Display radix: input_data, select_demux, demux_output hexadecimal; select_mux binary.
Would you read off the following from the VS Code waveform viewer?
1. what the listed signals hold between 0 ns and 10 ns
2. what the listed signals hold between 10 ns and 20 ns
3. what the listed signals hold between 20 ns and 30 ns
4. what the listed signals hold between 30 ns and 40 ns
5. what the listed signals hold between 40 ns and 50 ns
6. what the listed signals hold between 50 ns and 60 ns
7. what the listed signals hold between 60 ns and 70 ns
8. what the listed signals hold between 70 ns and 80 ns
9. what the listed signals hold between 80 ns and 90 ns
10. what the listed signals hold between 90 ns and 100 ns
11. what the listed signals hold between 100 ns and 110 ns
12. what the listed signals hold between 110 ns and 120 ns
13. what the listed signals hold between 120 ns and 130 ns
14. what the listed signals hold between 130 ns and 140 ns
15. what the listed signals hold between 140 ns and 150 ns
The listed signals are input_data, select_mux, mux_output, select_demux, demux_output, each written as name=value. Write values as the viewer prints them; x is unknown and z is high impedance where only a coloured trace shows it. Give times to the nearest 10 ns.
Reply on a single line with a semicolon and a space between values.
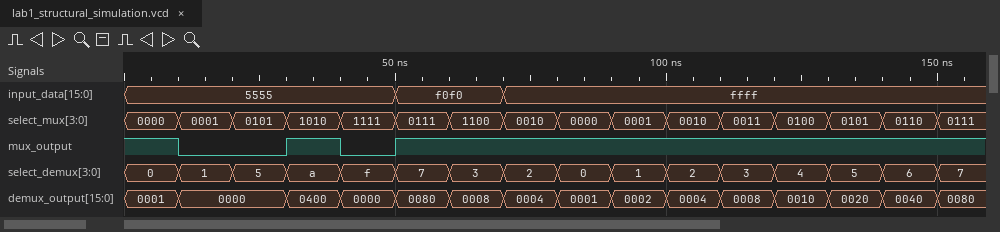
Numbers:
input_data=5555, select_mux=0000, mux_output=1, select_demux=0, demux_output=0001; input_data=5555, select_mux=0001, mux_output=0, select_demux=1, demux_output=0000; input_data=5555, select_mux=0101, mux_output=0, select_demux=5, demux_output=0000; input_data=5555, select_mux=1010, mux_output=1, select_demux=a, demux_output=0400; input_data=5555, select_mux=1111, mux_output=0, select_demux=f, demux_output=0000; input_data=f0f0, select_mux=0111, mux_output=1, select_demux=7, demux_output=0080; input_data=f0f0, select_mux=1100, mux_output=1, select_demux=3, demux_output=0008; input_data=ffff, select_mux=0010, mux_output=1, select_demux=2, demux_output=0004; input_data=ffff, select_mux=0000, mux_output=1, select_demux=0, demux_output=0001; input_data=ffff, select_mux=0001, mux_output=1, select_demux=1, demux_output=0002; input_data=ffff, select_mux=0010, mux_output=1, select_demux=2, demux_output=0004; input_data=ffff, select_mux=0011, mux_output=1, select_demux=3, demux_output=0008; input_data=ffff, select_mux=0100, mux_output=1, select_demux=4, demux_output=0010; input_data=ffff, select_mux=0101, mux_output=1, select_demux=5, demux_output=0020; input_data=ffff, select_mux=0110, mux_output=1, select_demux=6, demux_output=0040
